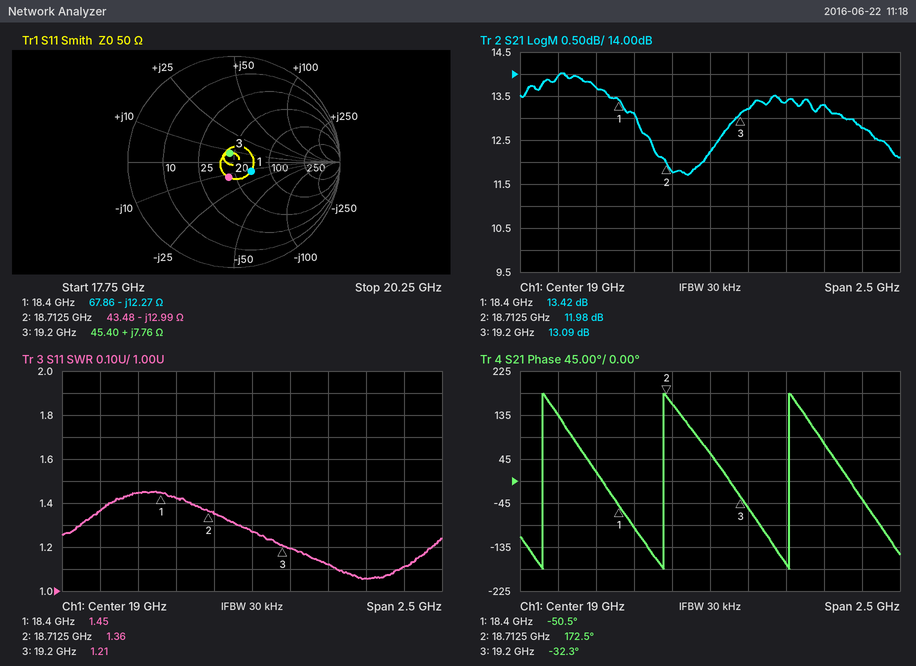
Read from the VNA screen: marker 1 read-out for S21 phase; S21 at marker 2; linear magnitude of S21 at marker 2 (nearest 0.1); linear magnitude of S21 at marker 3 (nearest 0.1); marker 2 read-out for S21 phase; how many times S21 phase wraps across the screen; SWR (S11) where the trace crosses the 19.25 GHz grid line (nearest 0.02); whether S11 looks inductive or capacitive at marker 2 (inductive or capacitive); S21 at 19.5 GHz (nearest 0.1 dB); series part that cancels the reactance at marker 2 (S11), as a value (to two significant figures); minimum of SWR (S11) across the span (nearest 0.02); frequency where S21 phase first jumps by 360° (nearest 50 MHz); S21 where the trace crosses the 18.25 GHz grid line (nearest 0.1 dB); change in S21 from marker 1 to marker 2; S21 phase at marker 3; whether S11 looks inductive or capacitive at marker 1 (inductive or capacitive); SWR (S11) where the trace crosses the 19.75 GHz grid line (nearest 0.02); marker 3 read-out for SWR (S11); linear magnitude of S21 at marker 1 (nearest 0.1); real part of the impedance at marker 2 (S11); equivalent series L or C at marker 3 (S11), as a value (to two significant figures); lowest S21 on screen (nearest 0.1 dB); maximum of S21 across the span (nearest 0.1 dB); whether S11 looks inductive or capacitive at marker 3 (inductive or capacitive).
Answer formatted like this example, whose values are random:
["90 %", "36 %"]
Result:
["-50.5°", "11.98 dB", "4.0", "4.5", "172.5°", "3", "1.20", "capacitive", "13.4 dB", "110 pH", "1.06", "17.90 GHz", "13.7 dB", "-1.44 dB", "-32.3°", "capacitive", "1.06", "1.21", "4.7", "43.48 Ω", "64 pH", "11.7 dB", "14.0 dB", "inductive"]
